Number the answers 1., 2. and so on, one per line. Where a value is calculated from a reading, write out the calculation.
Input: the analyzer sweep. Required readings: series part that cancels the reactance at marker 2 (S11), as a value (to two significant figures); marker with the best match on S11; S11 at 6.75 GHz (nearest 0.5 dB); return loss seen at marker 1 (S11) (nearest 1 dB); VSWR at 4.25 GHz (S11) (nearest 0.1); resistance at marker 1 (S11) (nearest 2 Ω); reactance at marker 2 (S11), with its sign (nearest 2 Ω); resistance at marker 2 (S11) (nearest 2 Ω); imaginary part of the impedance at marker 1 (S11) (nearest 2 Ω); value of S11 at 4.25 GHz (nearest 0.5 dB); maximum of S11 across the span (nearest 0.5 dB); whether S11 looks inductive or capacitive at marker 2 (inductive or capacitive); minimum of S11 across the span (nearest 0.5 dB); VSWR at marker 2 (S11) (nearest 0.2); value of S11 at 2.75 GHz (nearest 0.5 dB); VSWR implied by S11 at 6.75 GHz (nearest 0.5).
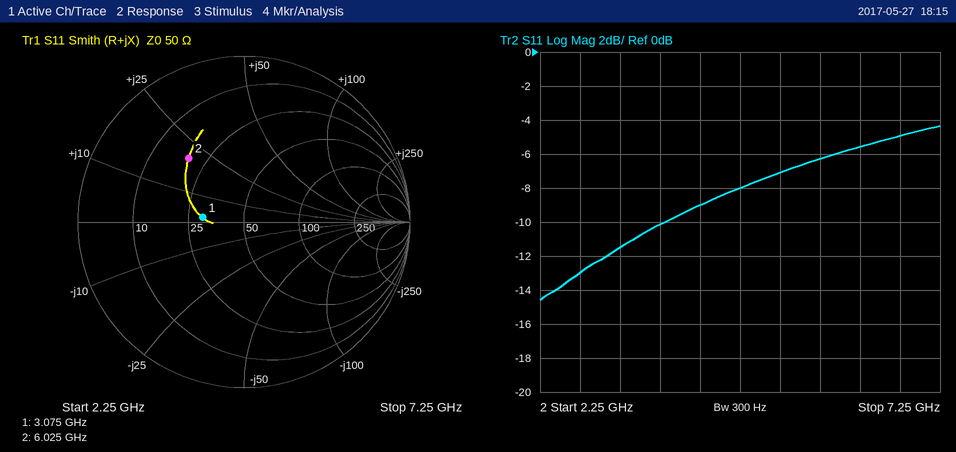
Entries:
1. C = 1/(2π × 6.025 GHz × 20 Ω) ≈ 1.3 pF
2. marker 1
3. -5.0 dB
4. 12 dB
5. |Γ| = 10^(-9/20) = 0.3548; VSWR = (1 + 0.3548)/(1 − 0.3548) ≈ 2.1
6. 30 Ω
7. +20 Ω
8. 20 Ω
9. +2 Ω
10. -9.0 dB
11. -4.5 dB
12. inductive
13. -14.5 dB
14. 3.0
15. -13.0 dB
16. |Γ| = 10^(-5/20) = 0.5623; VSWR = (1 + 0.5623)/(1 − 0.5623) ≈ 3.57, so 3.5 to the nearest 0.5
